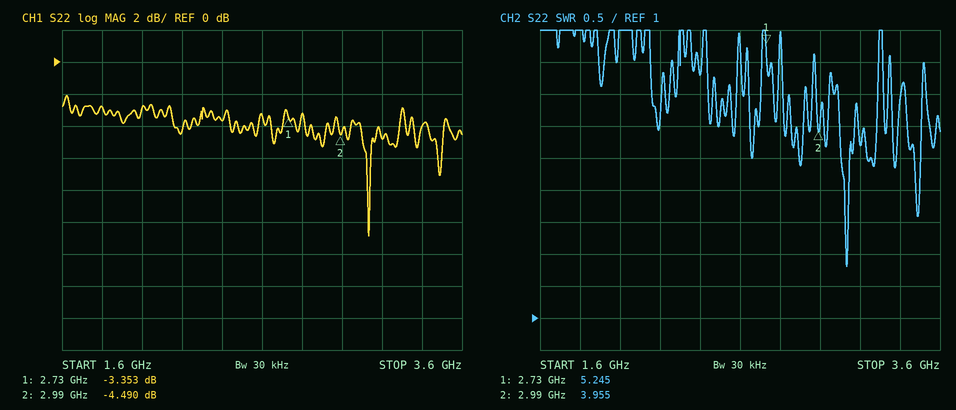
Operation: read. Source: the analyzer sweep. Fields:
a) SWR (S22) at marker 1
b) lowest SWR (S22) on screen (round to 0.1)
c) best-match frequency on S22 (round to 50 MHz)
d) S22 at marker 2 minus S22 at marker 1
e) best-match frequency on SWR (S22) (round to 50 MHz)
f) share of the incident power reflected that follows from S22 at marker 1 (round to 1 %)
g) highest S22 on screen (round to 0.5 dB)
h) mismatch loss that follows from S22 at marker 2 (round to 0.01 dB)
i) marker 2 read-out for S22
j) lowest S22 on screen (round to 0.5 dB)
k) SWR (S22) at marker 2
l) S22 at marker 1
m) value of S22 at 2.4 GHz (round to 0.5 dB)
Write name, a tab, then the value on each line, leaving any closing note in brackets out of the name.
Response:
SWR (S22) at marker 1	5.245
lowest SWR (S22) on screen	1.8
best-match frequency on S22	3.15 GHz
S22 at marker 2 minus S22 at marker 1	-1.137 dB
best-match frequency on SWR (S22)	3.15 GHz
share of the incident power reflected that follows from S22 at marker 1	46 %
highest S22 on screen	-2.0 dB
mismatch loss that follows from S22 at marker 2	1.91 dB
marker 2 read-out for S22	-4.490 dB
lowest S22 on screen	-11.0 dB
SWR (S22) at marker 2	3.955
S22 at marker 1	-3.353 dB
value of S22 at 2.4 GHz	-3.5 dB
